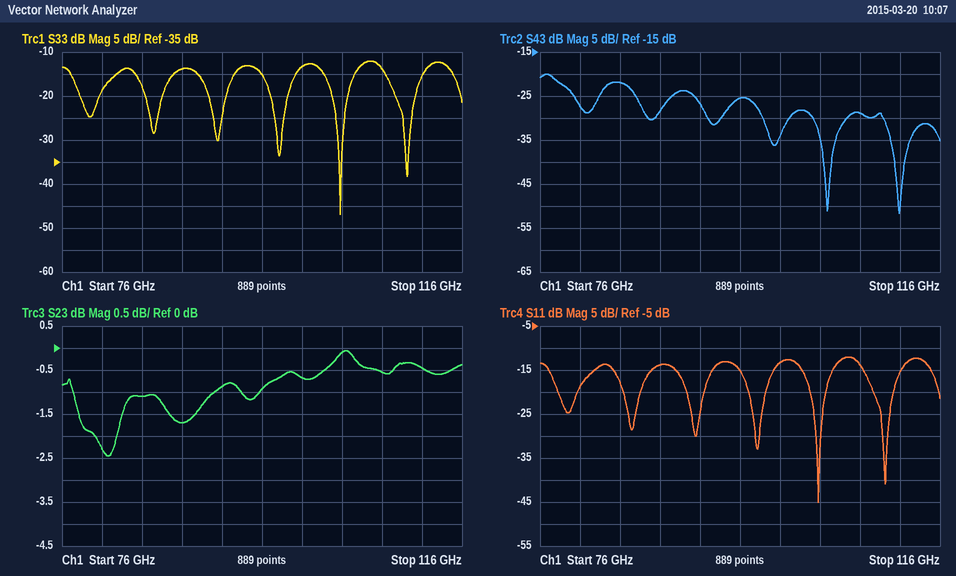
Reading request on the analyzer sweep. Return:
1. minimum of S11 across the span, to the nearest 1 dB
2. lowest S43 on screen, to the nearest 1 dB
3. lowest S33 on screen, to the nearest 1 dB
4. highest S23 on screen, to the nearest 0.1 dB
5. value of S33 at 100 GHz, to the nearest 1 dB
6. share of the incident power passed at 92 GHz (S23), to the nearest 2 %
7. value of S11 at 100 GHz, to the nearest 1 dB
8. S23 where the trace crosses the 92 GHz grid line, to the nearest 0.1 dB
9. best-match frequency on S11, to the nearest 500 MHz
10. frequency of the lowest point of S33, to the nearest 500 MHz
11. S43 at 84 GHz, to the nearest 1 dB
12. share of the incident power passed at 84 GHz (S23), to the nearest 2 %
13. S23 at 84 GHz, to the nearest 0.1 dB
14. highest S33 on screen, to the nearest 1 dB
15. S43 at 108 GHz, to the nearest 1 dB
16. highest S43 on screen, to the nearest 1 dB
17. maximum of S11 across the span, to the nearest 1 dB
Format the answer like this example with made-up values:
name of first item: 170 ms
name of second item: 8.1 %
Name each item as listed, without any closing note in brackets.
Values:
minimum of S11 across the span, to the nearest 1 dB: -45 dB
lowest S43 on screen, to the nearest 1 dB: -52 dB
lowest S33 on screen, to the nearest 1 dB: -47 dB
highest S23 on screen, to the nearest 0.1 dB: -0.1 dB
value of S33 at 100 GHz, to the nearest 1 dB: -13 dB
share of the incident power passed at 92 GHz (S23), to the nearest 2 %: 82 %
value of S11 at 100 GHz, to the nearest 1 dB: -13 dB
S23 where the trace crosses the 92 GHz grid line, to the nearest 0.1 dB: -0.9 dB
best-match frequency on S11, to the nearest 500 MHz: 104.0 GHz
frequency of the lowest point of S33, to the nearest 500 MHz: 104.0 GHz
S43 at 84 GHz, to the nearest 1 dB: -22 dB
share of the incident power passed at 84 GHz (S23), to the nearest 2 %: 78 %
S23 at 84 GHz, to the nearest 0.1 dB: -1.1 dB
highest S33 on screen, to the nearest 1 dB: -12 dB
S43 at 108 GHz, to the nearest 1 dB: -29 dB
highest S43 on screen, to the nearest 1 dB: -20 dB
maximum of S11 across the span, to the nearest 1 dB: -12 dB
